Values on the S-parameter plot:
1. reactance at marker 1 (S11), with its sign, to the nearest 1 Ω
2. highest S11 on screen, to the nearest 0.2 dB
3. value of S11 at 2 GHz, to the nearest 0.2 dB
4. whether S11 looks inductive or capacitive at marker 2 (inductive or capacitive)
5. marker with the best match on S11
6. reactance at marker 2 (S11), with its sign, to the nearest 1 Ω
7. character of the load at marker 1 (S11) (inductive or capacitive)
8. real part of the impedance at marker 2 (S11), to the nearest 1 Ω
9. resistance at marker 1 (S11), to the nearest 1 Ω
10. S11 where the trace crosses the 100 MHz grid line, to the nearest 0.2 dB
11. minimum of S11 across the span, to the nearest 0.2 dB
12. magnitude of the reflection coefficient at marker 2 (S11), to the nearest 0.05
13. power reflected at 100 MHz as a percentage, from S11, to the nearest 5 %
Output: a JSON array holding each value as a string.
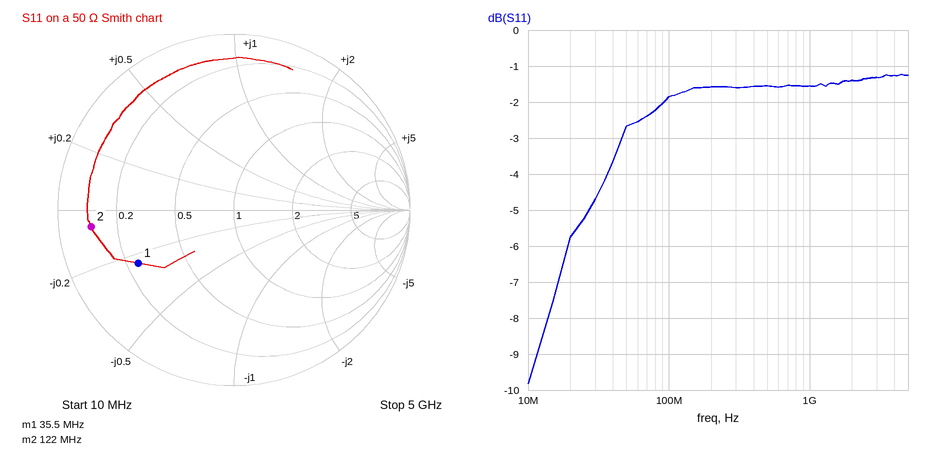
["-12 Ω", "-1.2 dB", "-1.4 dB", "capacitive", "marker 1", "-3 Ω", "capacitive", "5 Ω", "12 Ω", "-1.8 dB", "-9.8 dB", "0.80", "65 %"]
